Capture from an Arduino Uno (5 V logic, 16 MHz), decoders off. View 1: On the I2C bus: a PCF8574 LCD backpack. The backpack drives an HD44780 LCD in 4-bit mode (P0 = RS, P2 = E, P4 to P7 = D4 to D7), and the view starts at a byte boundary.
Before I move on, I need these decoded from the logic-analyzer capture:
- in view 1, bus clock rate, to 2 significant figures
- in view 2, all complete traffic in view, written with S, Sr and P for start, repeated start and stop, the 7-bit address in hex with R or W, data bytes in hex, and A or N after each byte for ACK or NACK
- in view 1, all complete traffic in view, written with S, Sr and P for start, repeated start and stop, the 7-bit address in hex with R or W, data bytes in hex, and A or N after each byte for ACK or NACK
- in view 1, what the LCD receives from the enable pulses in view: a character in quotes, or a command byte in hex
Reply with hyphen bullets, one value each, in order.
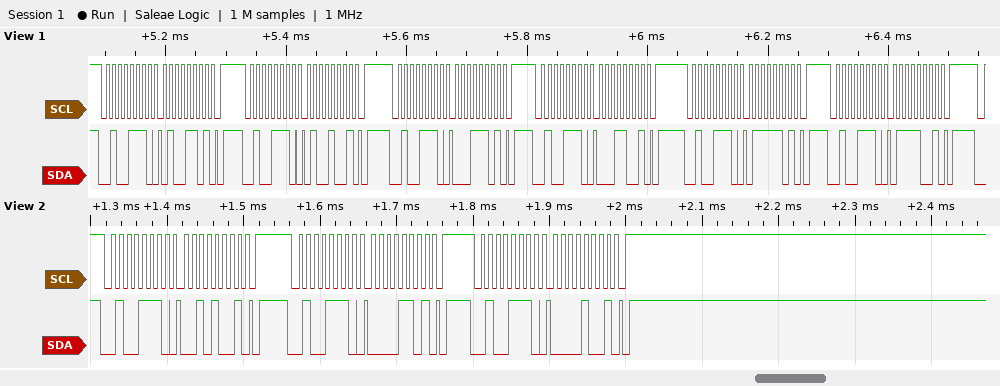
- 100 kHz
- S 27W A 29 A P S 27W A 0D A P S 27W A 09 A P
- S 27W A 4D A P S 27W A 49 A P S 27W A 1D A P S 27W A 19 A P S 27W A 7D A P S 27W A 79 A P
- 'A'
